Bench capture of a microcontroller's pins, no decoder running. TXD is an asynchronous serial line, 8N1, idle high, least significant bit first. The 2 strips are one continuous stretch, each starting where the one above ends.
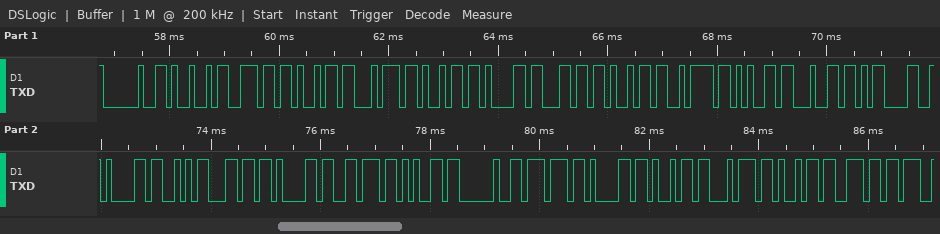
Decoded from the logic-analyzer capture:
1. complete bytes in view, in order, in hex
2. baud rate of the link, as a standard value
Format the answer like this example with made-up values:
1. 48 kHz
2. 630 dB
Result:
1. 0x20 0x49 0x6E 0x69 0x74 0x69 0x61 0x6C 0x69 0x7A 0x65 0x64 0x0D 0x0A 0x53 0x6C 0x61 0x76 0x65 0x20 0x77 0x61 0x69 0x74 0x69 0x6E
2. 9600 baud
